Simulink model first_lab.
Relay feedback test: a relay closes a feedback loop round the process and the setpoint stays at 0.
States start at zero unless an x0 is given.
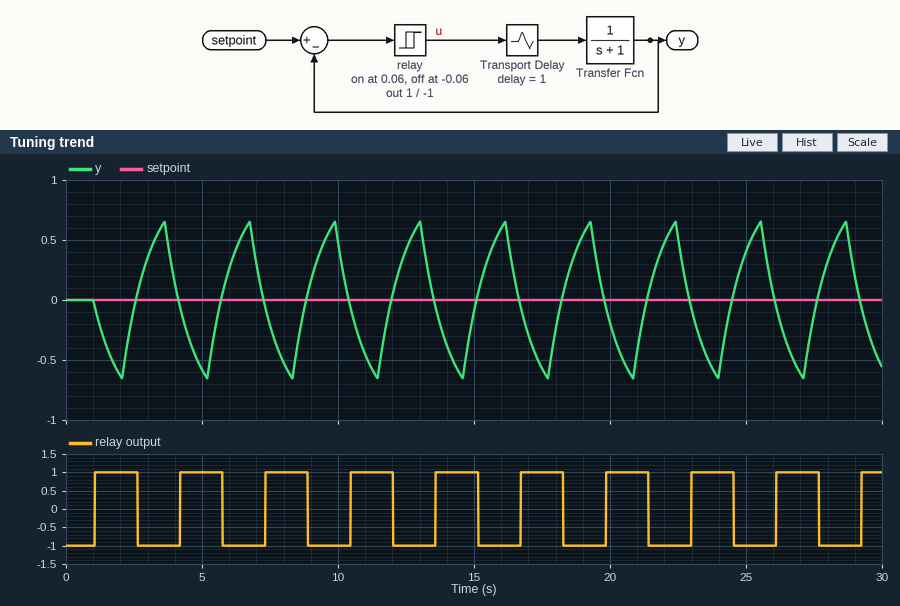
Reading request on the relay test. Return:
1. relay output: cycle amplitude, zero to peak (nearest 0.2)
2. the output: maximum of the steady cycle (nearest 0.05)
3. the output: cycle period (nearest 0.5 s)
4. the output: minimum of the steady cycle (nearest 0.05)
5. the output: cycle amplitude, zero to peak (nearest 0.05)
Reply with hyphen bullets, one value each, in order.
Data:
- 1.0
- 0.65
- 3.0 s
- -0.65
- 0.65
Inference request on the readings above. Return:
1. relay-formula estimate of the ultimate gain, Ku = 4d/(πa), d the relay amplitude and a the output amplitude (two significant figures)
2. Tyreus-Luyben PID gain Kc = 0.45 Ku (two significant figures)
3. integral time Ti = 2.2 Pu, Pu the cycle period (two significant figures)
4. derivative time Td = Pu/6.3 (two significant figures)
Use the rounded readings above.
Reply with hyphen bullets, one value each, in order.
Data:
- 2.0
- 0.90
- 6.6 s
- 0.48 s
